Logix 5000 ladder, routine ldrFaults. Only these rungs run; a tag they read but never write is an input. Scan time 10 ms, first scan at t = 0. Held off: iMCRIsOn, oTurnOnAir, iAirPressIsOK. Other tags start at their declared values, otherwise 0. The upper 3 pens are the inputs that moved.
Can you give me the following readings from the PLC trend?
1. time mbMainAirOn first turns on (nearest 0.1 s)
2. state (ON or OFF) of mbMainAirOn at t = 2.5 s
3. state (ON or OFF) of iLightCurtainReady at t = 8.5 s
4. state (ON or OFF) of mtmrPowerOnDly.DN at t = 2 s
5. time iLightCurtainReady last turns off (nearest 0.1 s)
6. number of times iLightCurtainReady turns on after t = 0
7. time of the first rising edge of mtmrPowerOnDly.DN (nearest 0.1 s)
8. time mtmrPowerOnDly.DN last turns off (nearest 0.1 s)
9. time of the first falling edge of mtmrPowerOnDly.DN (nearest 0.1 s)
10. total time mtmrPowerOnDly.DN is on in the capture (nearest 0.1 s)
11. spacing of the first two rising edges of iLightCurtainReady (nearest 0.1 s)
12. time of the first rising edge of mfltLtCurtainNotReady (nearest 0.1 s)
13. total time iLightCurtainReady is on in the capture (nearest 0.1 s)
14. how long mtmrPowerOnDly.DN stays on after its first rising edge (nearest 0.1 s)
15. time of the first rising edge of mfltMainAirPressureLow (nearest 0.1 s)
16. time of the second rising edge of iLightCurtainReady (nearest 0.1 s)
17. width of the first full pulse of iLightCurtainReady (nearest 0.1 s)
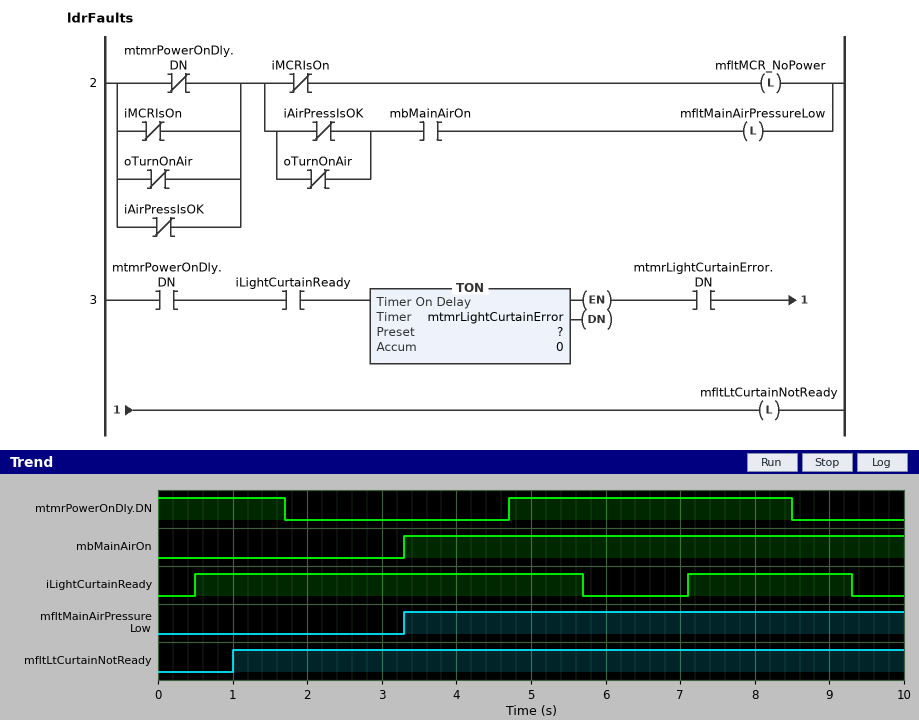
3.3 s
OFF
ON
OFF
9.3 s
2
4.7 s
8.5 s
1.7 s
5.5 s
6.6 s
1.0 s
7.4 s
3.8 s
3.3 s
7.1 s
5.2 s
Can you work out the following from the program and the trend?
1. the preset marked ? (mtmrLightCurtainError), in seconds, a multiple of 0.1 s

0.5 s
